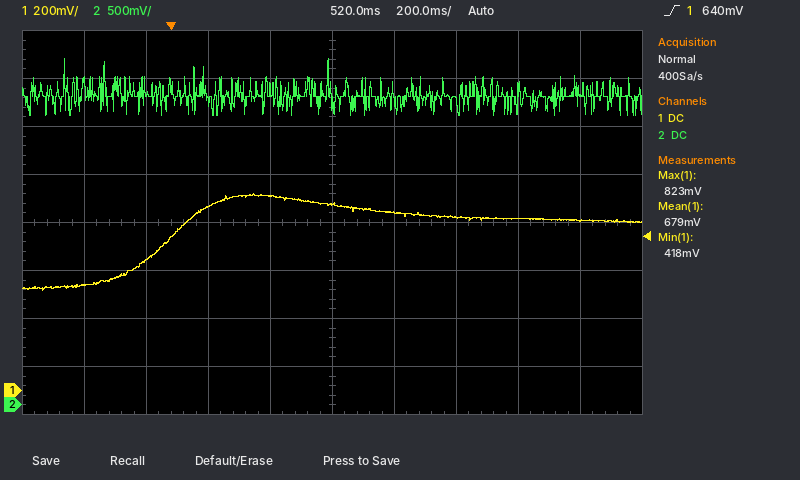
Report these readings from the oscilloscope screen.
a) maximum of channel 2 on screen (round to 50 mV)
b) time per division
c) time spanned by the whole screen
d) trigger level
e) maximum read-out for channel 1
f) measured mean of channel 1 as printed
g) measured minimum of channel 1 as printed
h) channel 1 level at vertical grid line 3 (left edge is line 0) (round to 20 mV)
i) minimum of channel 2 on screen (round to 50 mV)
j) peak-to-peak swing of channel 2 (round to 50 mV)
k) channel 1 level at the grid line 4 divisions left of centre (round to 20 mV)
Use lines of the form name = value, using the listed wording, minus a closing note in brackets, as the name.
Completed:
maximum of channel 2 on screen = 3.60 V
time per division = 200 ms
time spanned by the whole screen = 2 s
trigger level = 640 mV
maximum read-out for channel 1 = 823 mV
measured mean of channel 1 as printed = 679 mV
measured minimum of channel 1 as printed = 418 mV
channel 1 level at vertical grid line 3 (left edge is line 0) = 760 mV
minimum of channel 2 on screen = 3.00 V
peak-to-peak swing of channel 2 = 600 mV
channel 1 level at the grid line 4 divisions left of centre = 440 mV
